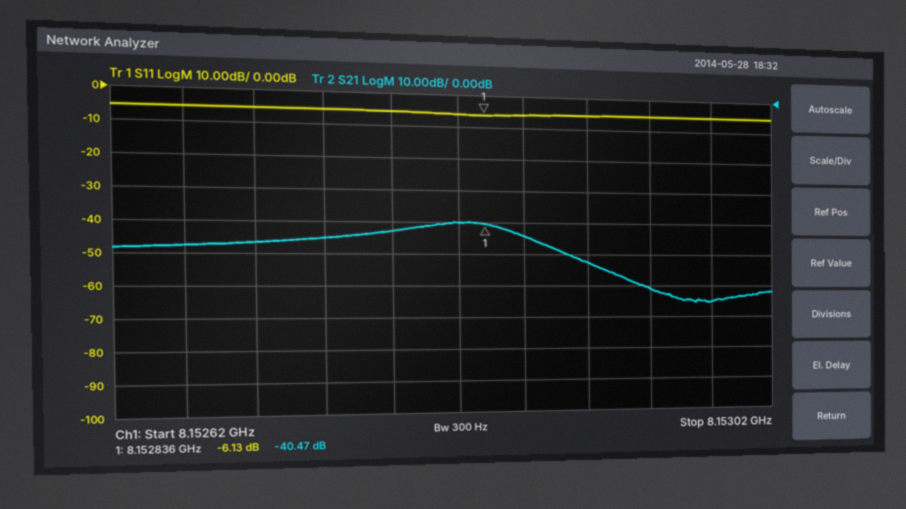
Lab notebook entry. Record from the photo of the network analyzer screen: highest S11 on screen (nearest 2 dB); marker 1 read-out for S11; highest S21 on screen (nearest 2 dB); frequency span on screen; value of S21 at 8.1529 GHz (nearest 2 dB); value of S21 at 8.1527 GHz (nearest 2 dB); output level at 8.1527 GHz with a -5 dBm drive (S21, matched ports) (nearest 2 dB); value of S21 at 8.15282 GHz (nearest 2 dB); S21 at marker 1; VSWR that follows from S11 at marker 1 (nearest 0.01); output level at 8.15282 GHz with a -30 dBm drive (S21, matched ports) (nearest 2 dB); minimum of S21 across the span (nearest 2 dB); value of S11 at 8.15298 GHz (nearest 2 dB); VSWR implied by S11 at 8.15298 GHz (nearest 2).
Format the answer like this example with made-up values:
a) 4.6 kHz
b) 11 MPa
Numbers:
a) -6 dB
b) -6.13 dB
c) -40 dB
d) 400 kHz
e) -52 dB
f) -46 dB
g) -52 dBm
h) -40 dB
i) -40.47 dB
j) 2.95
k) -70 dBm
l) -66 dB
m) -6 dB
n) 4
